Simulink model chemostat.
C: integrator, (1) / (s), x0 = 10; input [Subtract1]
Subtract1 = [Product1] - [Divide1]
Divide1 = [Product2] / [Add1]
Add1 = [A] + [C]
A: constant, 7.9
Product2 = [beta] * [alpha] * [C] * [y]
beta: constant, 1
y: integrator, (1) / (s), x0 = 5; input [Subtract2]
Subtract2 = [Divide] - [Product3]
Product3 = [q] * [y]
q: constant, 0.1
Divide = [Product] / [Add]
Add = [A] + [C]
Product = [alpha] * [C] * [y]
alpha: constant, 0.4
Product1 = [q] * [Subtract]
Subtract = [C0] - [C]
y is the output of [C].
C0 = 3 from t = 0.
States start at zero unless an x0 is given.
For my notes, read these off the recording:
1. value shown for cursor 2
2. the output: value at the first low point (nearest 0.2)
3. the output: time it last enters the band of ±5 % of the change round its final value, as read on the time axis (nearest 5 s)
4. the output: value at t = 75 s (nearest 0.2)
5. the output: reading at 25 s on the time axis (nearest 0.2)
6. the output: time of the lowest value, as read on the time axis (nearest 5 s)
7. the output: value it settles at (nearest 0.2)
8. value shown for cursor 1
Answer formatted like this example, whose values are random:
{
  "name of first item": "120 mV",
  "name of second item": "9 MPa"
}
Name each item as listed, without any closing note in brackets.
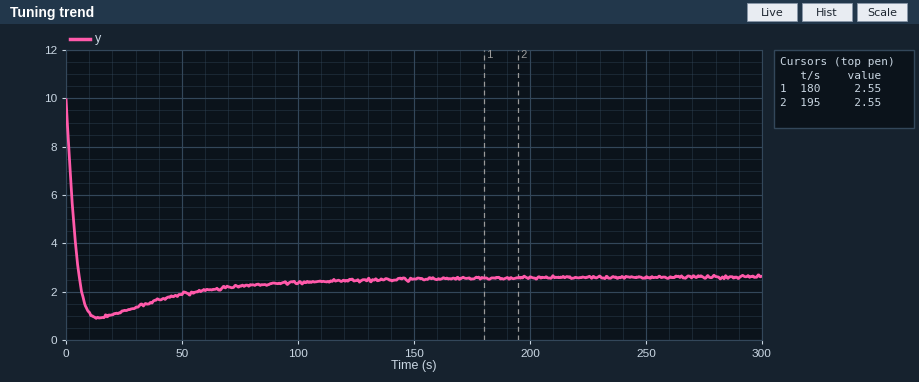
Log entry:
{
  "value shown for cursor 2": "2.55",
  "the output: value at the first low point": "1.0",
  "the output: time it last enters the band of ±5 % of the change round its final value, as read on the time axis": "80 s",
  "the output: value at t = 75 s": "2.2",
  "the output: reading at 25 s on the time axis": "1.2",
  "the output: time of the lowest value, as read on the time axis": "15 s",
  "the output: value it settles at": "2.6",
  "value shown for cursor 1": "2.55"
}
